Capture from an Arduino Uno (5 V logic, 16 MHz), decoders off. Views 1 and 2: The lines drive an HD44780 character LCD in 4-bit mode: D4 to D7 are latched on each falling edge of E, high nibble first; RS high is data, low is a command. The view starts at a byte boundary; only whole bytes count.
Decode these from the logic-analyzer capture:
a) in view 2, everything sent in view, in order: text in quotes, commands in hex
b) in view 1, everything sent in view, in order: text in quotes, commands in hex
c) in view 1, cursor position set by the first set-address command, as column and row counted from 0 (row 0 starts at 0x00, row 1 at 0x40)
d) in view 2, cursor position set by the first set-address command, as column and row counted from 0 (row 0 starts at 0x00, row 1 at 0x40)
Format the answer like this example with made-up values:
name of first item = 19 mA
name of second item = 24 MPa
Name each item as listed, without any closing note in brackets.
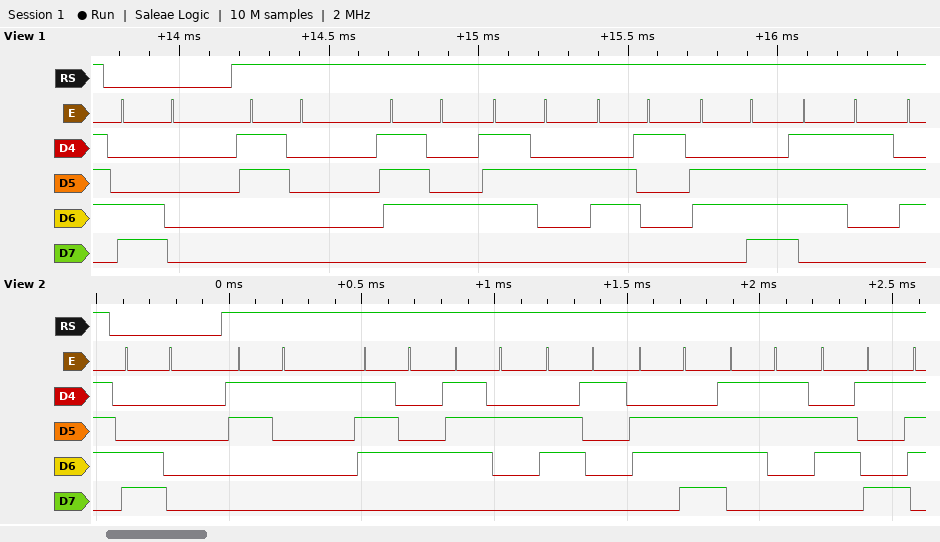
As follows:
in view 2, everything sent in view, in order: text in quotes, commands in hex = 0xC0 "1transi"
in view 1, everything sent in view, in order: text in quotes, commands in hex = 0xC0 "0trans"
in view 1, cursor position set by the first set-address command, as column and row counted from 0 = column 0, row 1
in view 2, cursor position set by the first set-address command, as column and row counted from 0 = column 0, row 1
